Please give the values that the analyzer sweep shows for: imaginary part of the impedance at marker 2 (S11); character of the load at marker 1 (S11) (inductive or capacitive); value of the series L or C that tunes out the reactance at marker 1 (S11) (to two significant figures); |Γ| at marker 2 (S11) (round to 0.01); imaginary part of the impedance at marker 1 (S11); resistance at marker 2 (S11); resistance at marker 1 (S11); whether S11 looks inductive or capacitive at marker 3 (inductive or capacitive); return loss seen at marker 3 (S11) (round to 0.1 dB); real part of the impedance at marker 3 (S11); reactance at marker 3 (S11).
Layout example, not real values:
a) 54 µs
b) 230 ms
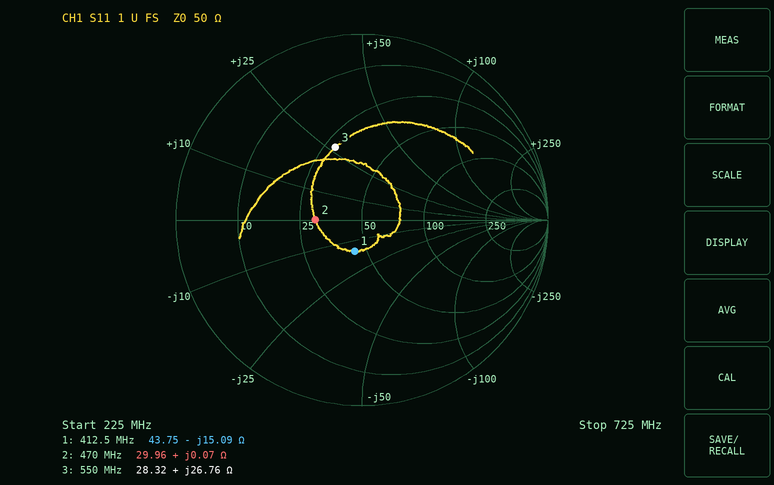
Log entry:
a) +0.07 Ω
b) capacitive
c) 5.8 nH
d) 0.25
e) -15.09 Ω
f) 29.96 Ω
g) 43.75 Ω
h) inductive
i) 7.6 dB
j) 28.32 Ω
k) +26.76 Ω
